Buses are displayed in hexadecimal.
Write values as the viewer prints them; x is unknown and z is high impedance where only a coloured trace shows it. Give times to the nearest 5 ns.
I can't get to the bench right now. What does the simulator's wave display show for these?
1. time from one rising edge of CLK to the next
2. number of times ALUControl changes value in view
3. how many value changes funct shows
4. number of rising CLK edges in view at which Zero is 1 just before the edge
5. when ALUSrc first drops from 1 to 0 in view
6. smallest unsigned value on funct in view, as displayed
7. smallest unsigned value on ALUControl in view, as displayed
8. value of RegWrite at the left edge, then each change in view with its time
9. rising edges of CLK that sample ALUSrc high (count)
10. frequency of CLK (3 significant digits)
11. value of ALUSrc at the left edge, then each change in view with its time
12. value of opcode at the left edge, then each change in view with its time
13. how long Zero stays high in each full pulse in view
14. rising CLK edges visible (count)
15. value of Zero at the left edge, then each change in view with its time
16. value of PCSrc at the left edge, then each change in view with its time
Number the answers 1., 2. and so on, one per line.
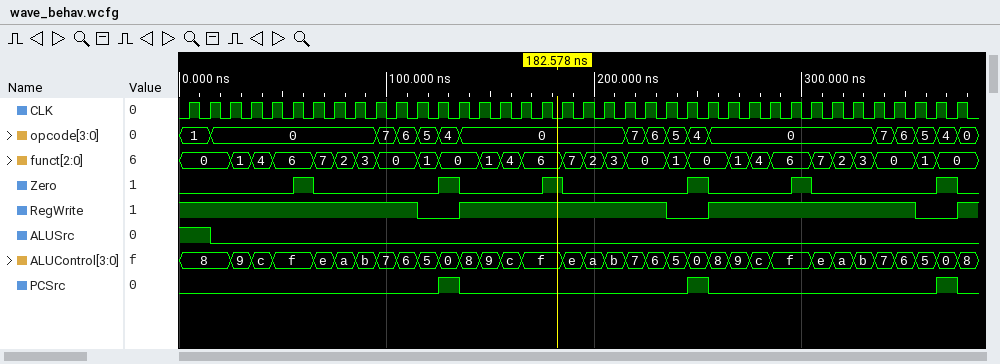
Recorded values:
1. 10 ns
2. 33
3. 27
4. 6
5. 15 ns
6. 0
7. 0
8. 1, 0 at 115 ns, 1 at 135 ns, 0 at 235 ns, 1 at 255 ns, 0 at 355 ns, 1 at 375 ns
9. 2
10. 100 MHz
11. 1, 0 at 15 ns
12. 1, 0 at 15 ns, 7 at 95 ns, 6 at 105 ns, 5 at 115 ns, 4 at 125 ns, 0 at 135 ns, 7 at 215 ns, 6 at 225 ns, 5 at 235 ns, 4 at 245 ns, 0 at 255 ns, 7 at 335 ns, 6 at 345 ns, 5 at 355 ns, 4 at 365 ns, 0 at 375 ns
13. 10 ns, 10 ns, 10 ns, 10 ns, 10 ns, 10 ns
14. 38
15. 0, 1 at 55 ns, 0 at 65 ns, 1 at 125 ns, 0 at 135 ns, 1 at 175 ns, 0 at 185 ns, 1 at 245 ns, 0 at 255 ns, 1 at 295 ns, 0 at 305 ns, 1 at 365 ns, 0 at 375 ns
16. 0, 1 at 125 ns, 0 at 135 ns, 1 at 245 ns, 0 at 255 ns, 1 at 365 ns, 0 at 375 ns
